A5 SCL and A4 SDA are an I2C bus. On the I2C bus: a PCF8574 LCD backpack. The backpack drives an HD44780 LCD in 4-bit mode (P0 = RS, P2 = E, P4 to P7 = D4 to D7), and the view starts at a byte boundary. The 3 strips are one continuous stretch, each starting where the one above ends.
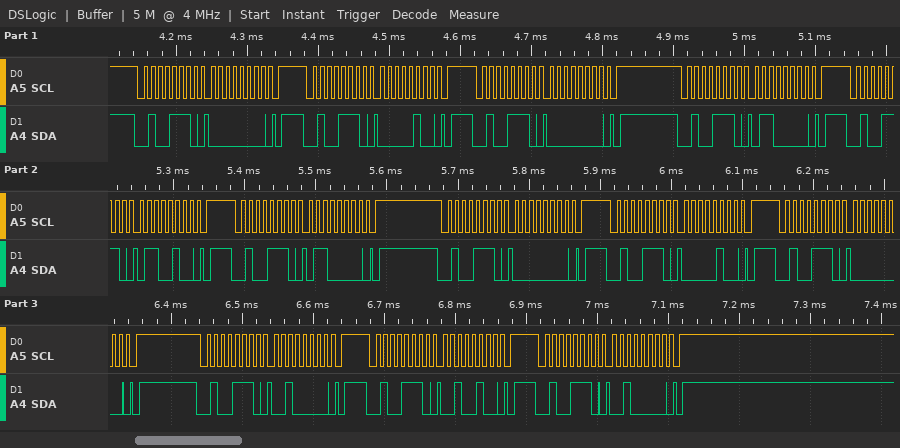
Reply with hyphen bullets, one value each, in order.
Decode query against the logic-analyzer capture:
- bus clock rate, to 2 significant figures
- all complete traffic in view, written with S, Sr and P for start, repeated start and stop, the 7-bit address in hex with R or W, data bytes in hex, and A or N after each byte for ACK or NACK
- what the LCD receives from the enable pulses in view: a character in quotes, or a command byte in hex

- 100 kHz
- S 27W A 00 A P S 27W A 04 A P S 27W A 00 A P S 27W A 60 A P S 27W A 64 A P S 27W A 60 A P S 27W A 00 A P S 27W A 04 A P S 27W A 00 A P S 27W A 20 A P S 27W A 24 A P S 27W A 20 A P
- 0x06 0x02
